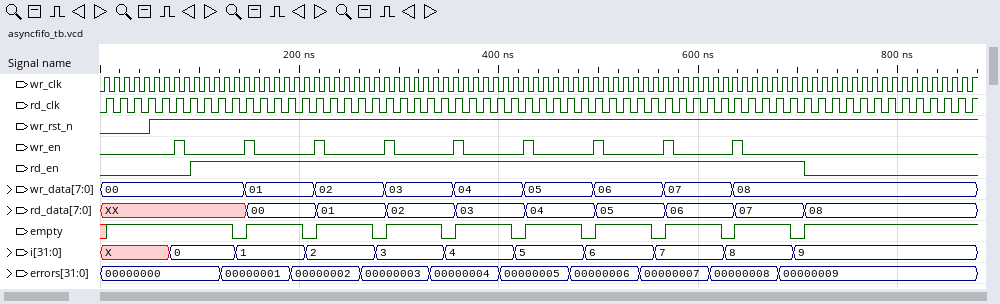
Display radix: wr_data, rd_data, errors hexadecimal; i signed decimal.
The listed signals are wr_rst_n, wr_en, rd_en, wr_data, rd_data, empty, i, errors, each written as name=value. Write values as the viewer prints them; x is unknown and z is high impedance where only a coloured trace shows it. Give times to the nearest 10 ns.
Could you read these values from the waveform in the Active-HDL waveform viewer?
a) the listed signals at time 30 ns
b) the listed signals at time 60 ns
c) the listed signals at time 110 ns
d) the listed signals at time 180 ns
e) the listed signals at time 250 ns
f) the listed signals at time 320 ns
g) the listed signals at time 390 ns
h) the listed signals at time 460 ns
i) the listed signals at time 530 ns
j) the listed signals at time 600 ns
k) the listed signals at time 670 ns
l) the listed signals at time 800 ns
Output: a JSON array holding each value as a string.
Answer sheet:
["wr_rst_n=0, wr_en=0, rd_en=0, wr_data=00, rd_data=XX, empty=1, i=X, errors=00000000", "wr_rst_n=1, wr_en=0, rd_en=0, wr_data=00, rd_data=XX, empty=1, i=X, errors=00000000", "wr_rst_n=1, wr_en=0, rd_en=1, wr_data=00, rd_data=XX, empty=1, i=0, errors=00000000", "wr_rst_n=1, wr_en=0, rd_en=1, wr_data=01, rd_data=00, empty=1, i=1, errors=00000001", "wr_rst_n=1, wr_en=0, rd_en=1, wr_data=02, rd_data=01, empty=1, i=2, errors=00000002", "wr_rst_n=1, wr_en=0, rd_en=1, wr_data=03, rd_data=02, empty=1, i=3, errors=00000003", "wr_rst_n=1, wr_en=0, rd_en=1, wr_data=04, rd_data=03, empty=1, i=4, errors=00000004", "wr_rst_n=1, wr_en=0, rd_en=1, wr_data=05, rd_data=04, empty=1, i=5, errors=00000005", "wr_rst_n=1, wr_en=0, rd_en=1, wr_data=06, rd_data=05, empty=1, i=6, errors=00000006", "wr_rst_n=1, wr_en=0, rd_en=1, wr_data=07, rd_data=06, empty=1, i=7, errors=00000007", "wr_rst_n=1, wr_en=0, rd_en=1, wr_data=08, rd_data=07, empty=1, i=8, errors=00000008", "wr_rst_n=1, wr_en=0, rd_en=0, wr_data=08, rd_data=08, empty=1, i=9, errors=00000009"]
